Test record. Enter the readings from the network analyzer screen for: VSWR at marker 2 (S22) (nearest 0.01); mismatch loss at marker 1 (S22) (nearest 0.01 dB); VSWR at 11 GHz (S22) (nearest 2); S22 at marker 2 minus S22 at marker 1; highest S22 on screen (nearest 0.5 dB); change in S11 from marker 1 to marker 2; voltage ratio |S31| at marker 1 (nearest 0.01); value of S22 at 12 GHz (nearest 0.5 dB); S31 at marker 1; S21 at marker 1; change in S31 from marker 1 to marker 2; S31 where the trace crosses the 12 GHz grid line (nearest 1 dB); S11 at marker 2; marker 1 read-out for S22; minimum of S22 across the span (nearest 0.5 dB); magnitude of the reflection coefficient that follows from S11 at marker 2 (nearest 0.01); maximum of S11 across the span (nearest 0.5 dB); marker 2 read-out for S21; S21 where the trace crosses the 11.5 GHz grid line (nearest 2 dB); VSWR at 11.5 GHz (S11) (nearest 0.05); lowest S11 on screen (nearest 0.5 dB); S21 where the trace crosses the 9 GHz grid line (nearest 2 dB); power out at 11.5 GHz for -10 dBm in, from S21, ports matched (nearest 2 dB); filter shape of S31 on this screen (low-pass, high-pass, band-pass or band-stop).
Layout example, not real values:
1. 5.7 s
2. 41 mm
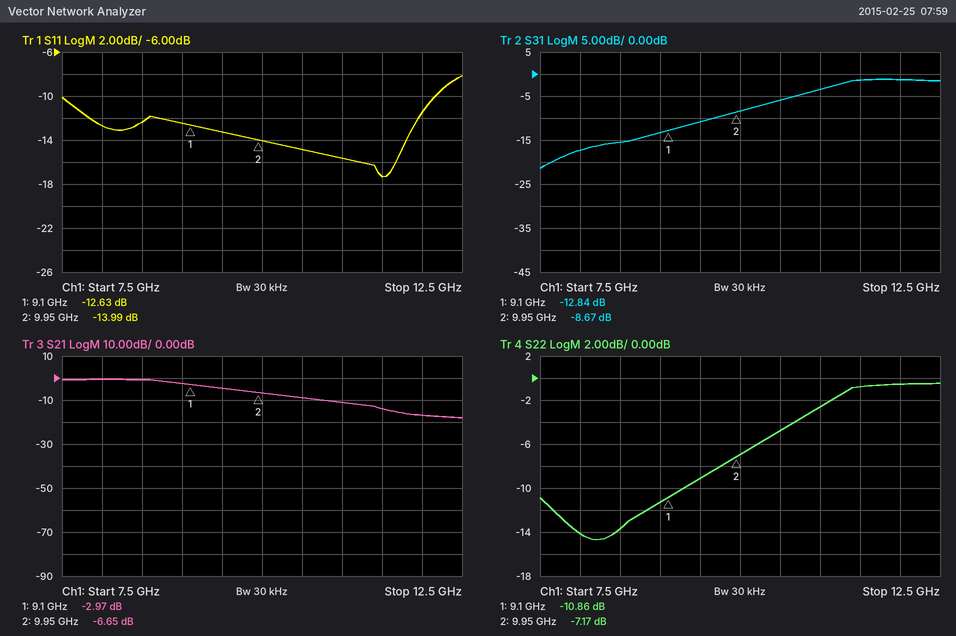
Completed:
1. 2.56
2. 0.37 dB
3. 6
4. 3.69 dB
5. -0.5 dB
6. -1.36 dB
7. 0.23
8. -0.5 dB
9. -12.84 dB
10. -2.97 dB
11. 4.17 dB
12. -1 dB
13. -13.99 dB
14. -10.86 dB
15. -14.5 dB
16. 0.20
17. -8.0 dB
18. -6.65 dB
19. -14 dB
20. 1.30
21. -17.5 dB
22. -2 dB
23. -24 dBm
24. high-pass
